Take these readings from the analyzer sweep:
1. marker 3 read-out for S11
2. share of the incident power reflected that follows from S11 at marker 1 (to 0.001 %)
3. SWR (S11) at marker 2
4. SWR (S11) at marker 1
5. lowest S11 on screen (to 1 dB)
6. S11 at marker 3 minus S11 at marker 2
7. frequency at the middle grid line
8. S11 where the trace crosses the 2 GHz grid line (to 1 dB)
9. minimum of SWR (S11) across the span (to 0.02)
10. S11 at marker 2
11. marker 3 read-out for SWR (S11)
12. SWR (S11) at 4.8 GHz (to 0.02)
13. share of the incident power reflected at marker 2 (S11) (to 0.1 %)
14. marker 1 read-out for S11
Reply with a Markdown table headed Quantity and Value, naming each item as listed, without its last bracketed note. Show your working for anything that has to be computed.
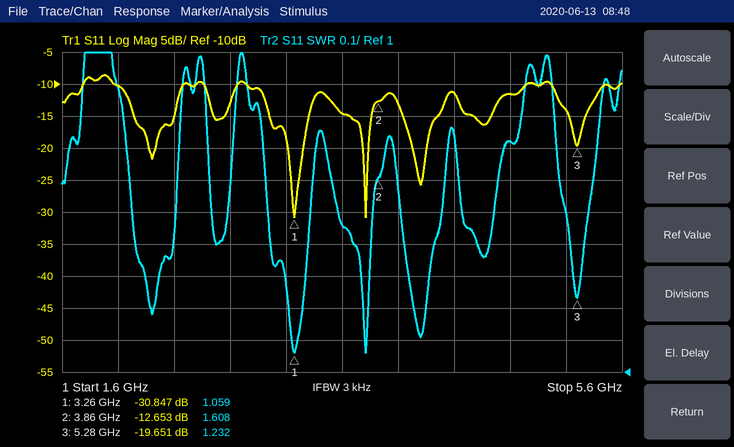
| Quantity | Value |
|---|---|
| marker 3 read-out for S11 | -19.651 dB |
| share of the incident power reflected that follows from S11 at marker 1 | 10^(-30.847/10) ≈ 0.082 % |
| SWR (S11) at marker 2 | 1.608 |
| SWR (S11) at marker 1 | 1.059 |
| lowest S11 on screen | -31 dB |
| S11 at marker 3 minus S11 at marker 2 | -19.651 − (-12.653) = -6.998 dB |
| frequency at the middle grid line | 3.6 GHz |
| S11 where the trace crosses the 2 GHz grid line | -10 dB |
| minimum of SWR (S11) across the span | 1.06 |
| S11 at marker 2 | -12.653 dB |
| marker 3 read-out for SWR | 1.232 |
| SWR (S11) at 4.8 GHz | 1.72 |
| share of the incident power reflected at marker 2 (S11) | 10^(-12.653/10) ≈ 5.4 % |
| marker 1 read-out for S11 | -30.847 dB |
